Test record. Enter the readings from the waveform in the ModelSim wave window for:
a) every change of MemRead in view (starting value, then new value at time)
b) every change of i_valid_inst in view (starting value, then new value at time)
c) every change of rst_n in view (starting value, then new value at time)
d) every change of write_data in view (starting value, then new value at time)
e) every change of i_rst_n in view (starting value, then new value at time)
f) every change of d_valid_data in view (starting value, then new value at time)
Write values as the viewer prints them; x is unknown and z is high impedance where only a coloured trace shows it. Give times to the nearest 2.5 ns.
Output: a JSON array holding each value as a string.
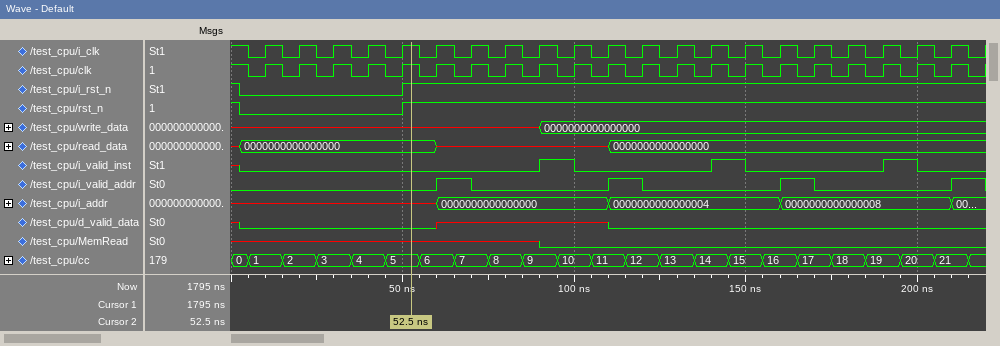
["x, 0 at 90 ns", "x, 0 at 2.5 ns, 1 at 90 ns, 0 at 100 ns, 1 at 140 ns, 0 at 150 ns, 1 at 190 ns, 0 at 200 ns", "1, 0 at 2.5 ns, 1 at 50 ns", "x, 0000000000000000 at 90 ns", "1, 0 at 2.5 ns, 1 at 50 ns", "x, 0 at 2.5 ns, x at 60 ns, 0 at 110 ns"]
